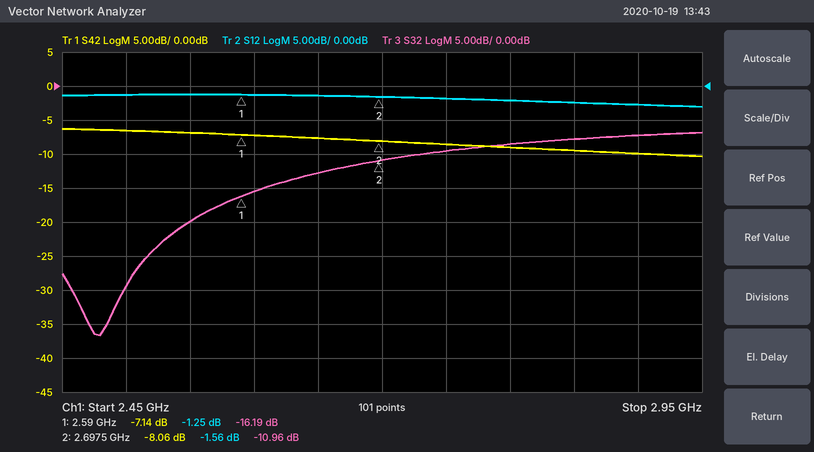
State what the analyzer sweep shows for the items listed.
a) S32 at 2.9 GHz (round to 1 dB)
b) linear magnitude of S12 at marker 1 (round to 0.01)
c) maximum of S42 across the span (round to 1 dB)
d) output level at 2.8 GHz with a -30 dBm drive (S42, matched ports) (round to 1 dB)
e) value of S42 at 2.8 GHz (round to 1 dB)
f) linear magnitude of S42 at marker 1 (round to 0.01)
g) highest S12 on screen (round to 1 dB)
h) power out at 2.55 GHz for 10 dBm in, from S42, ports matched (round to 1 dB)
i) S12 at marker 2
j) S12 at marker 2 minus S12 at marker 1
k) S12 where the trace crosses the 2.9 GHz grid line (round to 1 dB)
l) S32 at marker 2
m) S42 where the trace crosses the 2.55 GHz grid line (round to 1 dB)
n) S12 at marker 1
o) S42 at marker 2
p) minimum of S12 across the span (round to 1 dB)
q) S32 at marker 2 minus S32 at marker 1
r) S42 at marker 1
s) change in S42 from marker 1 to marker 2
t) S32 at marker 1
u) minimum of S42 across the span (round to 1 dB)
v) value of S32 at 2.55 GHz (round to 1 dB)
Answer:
-7 dB
0.87
-6 dB
-39 dBm
-9 dB
0.44
-1 dB
3 dBm
-1.56 dB
-0.31 dB
-3 dB
-10.96 dB
-7 dB
-1.25 dB
-8.06 dB
-3 dB
5.23 dB
-7.14 dB
-0.92 dB
-16.19 dB
-10 dB
-20 dB
